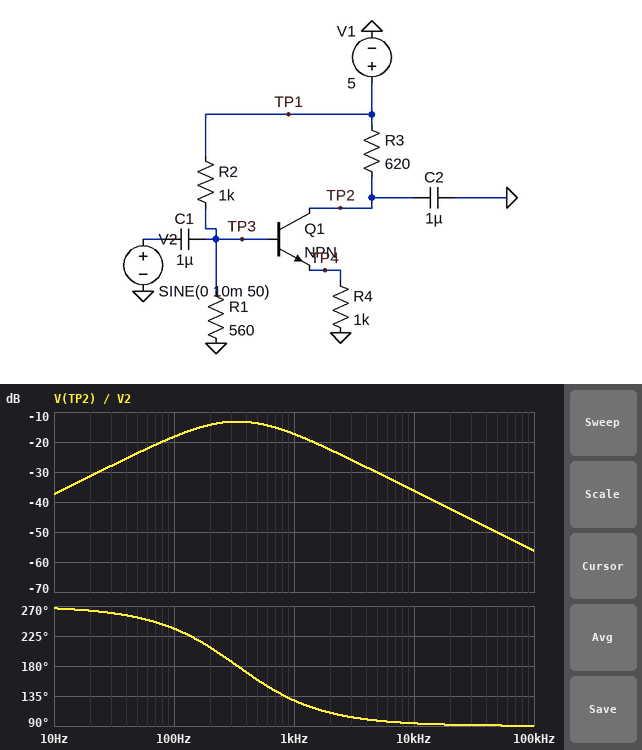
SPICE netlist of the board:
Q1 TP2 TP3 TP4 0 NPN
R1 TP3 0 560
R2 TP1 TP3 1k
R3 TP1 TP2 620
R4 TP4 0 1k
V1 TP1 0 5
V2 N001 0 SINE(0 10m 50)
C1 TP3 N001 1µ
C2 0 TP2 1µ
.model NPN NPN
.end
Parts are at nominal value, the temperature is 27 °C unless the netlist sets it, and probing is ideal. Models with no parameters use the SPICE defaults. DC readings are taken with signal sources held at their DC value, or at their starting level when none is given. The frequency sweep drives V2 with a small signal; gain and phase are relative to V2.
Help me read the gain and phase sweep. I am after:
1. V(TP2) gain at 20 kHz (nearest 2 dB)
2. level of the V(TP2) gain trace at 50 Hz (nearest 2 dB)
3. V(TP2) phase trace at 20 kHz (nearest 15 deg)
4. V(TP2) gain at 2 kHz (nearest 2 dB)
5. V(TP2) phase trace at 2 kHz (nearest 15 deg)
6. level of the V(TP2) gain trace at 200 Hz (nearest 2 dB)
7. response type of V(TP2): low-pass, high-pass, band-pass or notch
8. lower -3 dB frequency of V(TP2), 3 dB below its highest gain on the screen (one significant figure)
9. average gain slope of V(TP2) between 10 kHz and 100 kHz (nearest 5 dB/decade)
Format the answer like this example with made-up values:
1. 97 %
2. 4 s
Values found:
1. -42 dB
2. -24 dB
3. 90 deg
4. -22 dB
5. 105 deg
6. -14 dB
7. band-pass
8. 100 Hz
9. -20 dB/decade
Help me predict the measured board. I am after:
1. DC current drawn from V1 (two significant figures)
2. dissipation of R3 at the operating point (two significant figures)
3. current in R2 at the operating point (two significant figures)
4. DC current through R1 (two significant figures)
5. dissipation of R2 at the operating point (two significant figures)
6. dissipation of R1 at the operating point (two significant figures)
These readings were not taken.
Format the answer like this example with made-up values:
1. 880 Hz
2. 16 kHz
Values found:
1. 4.2 mA
2. 630 µW
3. 3.2 mA
4. 3.2 mA
5. 10 mW
6. 5.7 mW
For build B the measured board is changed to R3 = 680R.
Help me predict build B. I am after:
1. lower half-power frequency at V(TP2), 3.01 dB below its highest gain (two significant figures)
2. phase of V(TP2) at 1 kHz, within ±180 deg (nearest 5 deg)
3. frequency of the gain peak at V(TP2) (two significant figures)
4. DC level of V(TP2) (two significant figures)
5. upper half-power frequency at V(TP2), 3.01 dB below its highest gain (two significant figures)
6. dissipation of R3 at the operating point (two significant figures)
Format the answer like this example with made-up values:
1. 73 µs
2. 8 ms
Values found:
1. 130 Hz
2. 125 deg
3. 320 Hz
4. 4.3 V
5. 810 Hz
6. 690 µW
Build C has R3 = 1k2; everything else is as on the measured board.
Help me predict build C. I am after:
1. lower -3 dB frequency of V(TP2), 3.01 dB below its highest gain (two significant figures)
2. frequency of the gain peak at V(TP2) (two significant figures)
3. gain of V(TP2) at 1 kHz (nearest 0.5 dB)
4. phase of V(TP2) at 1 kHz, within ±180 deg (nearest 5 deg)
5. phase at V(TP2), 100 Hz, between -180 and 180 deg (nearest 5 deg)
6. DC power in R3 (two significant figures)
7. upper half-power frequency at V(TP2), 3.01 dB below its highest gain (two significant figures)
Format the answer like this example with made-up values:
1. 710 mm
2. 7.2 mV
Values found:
1. 89 Hz
2. 240 Hz
3. -17.0 dB
4. 120 deg
5. -140 deg
6. 1.2 mW
7. 670 Hz
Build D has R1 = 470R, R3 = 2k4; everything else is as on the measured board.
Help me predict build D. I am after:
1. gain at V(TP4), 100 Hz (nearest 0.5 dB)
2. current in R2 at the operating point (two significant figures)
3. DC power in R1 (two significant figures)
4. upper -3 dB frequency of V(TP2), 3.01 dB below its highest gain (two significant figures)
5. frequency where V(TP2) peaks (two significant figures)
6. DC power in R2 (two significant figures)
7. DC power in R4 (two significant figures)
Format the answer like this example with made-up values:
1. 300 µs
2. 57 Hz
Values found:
1. -14.5 dB
2. 3.4 mA
3. 5.4 mW
4. 620 Hz
5. 180 Hz
6. 12 mW
7. 680 µW
